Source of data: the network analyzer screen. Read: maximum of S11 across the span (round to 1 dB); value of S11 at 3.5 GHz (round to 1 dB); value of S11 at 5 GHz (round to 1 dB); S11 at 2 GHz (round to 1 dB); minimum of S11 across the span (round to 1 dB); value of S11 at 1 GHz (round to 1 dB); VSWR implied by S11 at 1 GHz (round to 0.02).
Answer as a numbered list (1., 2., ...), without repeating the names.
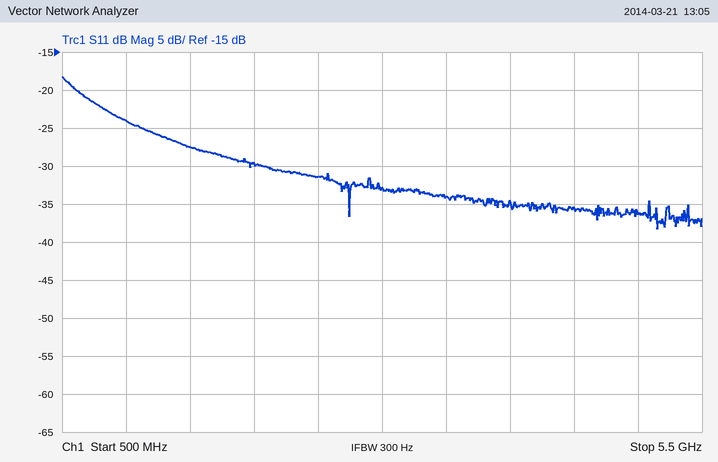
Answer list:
1. -18 dB
2. -34 dB
3. -36 dB
4. -30 dB
5. -38 dB
6. -24 dB
7. 1.14
